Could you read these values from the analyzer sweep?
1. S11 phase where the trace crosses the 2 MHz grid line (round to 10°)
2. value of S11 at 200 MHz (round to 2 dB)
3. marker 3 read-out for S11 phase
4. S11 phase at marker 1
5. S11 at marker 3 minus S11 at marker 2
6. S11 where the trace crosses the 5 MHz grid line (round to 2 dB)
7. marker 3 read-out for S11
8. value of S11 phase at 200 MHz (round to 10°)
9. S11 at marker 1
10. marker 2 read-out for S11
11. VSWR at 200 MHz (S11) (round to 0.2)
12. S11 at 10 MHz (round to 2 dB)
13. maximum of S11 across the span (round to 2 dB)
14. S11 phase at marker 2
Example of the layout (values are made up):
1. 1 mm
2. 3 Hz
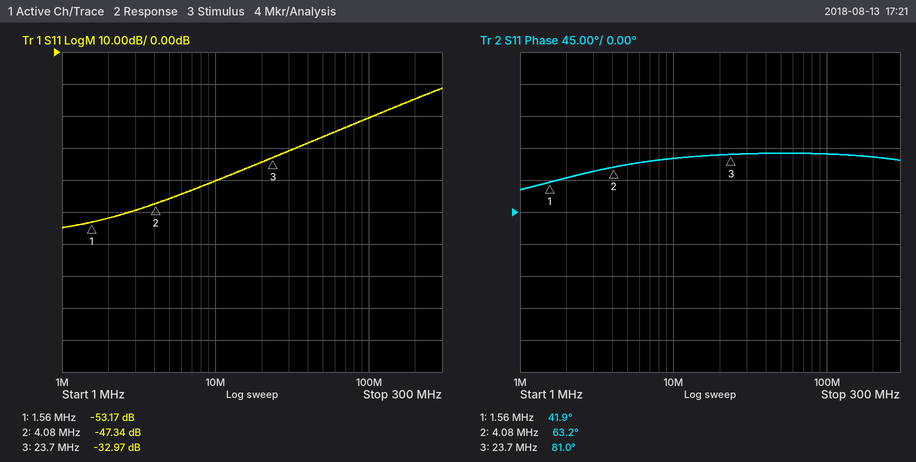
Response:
1. 50°
2. -14 dB
3. 81.0°
4. 41.9°
5. 14.37 dB
6. -46 dB
7. -32.97 dB
8. 80°
9. -53.17 dB
10. -47.34 dB
11. 1.4
12. -40 dB
13. -12 dB
14. 63.2°
